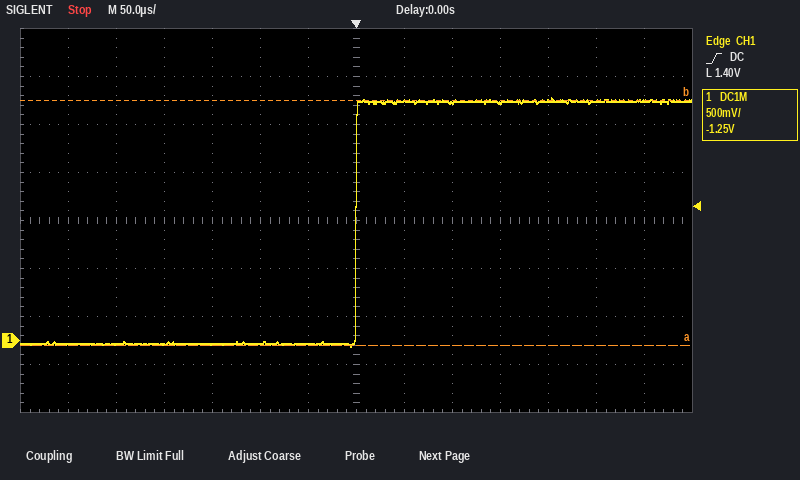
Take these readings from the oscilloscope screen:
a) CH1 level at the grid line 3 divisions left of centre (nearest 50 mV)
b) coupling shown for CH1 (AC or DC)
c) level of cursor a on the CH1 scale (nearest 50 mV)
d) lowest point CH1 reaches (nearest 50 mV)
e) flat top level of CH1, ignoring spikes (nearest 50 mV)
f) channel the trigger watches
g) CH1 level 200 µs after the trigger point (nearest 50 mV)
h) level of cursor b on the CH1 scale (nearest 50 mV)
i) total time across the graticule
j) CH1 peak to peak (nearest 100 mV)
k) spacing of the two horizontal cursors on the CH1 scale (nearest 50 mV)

-50 mV
DC
-50 mV
-50 mV
2.50 V
CH1
2.50 V
2.50 V
700 µs
2.60 V
2.55 V
